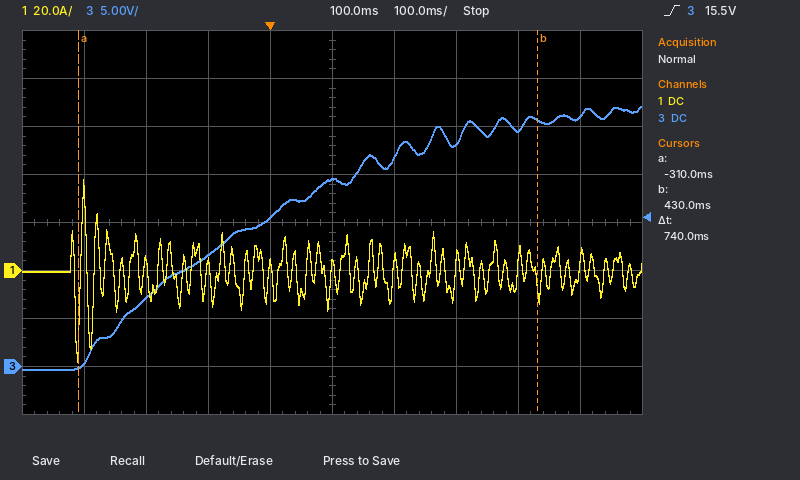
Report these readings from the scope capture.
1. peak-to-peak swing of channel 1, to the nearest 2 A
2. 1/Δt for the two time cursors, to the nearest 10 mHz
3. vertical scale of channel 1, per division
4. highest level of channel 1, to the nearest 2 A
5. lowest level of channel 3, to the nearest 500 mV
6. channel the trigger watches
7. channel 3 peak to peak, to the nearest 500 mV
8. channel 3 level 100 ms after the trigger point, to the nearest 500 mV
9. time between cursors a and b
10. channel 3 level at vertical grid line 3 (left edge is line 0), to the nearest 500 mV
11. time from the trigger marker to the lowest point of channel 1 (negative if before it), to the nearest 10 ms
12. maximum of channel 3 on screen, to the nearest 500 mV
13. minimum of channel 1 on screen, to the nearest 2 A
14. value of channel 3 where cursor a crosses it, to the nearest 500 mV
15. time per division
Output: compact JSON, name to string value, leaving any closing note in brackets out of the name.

{"peak-to-peak swing of channel 1, to the nearest 2 A": "76 A", "1/Δt for the two time cursors, to the nearest 10 mHz": "1.35 Hz", "vertical scale of channel 1, per division": "20 A", "highest level of channel 1, to the nearest 2 A": "38 A", "lowest level of channel 3, to the nearest 500 mV": "-500 mV", "channel the trigger watches": "channel 3", "channel 3 peak to peak, to the nearest 500 mV": "27.5 V", "channel 3 level 100 ms after the trigger point, to the nearest 500 mV": "19.5 V", "time between cursors a and b": "740 ms", "channel 3 level at vertical grid line 3 (left edge is line 0), to the nearest 500 mV": "11.5 V", "time from the trigger marker to the lowest point of channel 1 (negative if before it), to the nearest 10 ms": "-310 ms", "maximum of channel 3 on screen, to the nearest 500 mV": "27.0 V", "minimum of channel 1 on screen, to the nearest 2 A": "-38 A", "value of channel 3 where cursor a crosses it, to the nearest 500 mV": "0.0 V", "time per division": "100 ms"}
